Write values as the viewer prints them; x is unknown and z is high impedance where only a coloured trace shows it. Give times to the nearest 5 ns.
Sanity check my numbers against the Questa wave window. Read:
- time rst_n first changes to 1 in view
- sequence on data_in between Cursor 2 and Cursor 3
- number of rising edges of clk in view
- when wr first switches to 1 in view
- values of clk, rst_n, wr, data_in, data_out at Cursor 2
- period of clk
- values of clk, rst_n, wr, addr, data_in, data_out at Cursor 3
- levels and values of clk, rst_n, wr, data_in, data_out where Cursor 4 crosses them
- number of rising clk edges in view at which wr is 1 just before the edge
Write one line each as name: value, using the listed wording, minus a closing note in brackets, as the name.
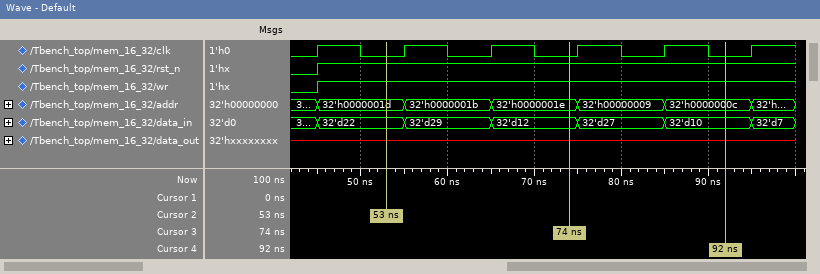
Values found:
time rst_n first changes to 1 in view: 45 ns
sequence on data_in between Cursor 2 and Cursor 3: 32'd22, 32'd29, 32'd12
number of rising edges of clk in view: 6
when wr first switches to 1 in view: 45 ns
values of clk, rst_n, wr, data_in, data_out at Cursor 2: clk=0, rst_n=1, wr=1, data_in=32'd22, data_out=x
period of clk: 10 ns
values of clk, rst_n, wr, addr, data_in, data_out at Cursor 3: clk=0, rst_n=1, wr=1, addr=32'h0000001e, data_in=32'd12, data_out=x
levels and values of clk, rst_n, wr, data_in, data_out where Cursor 4 crosses them: clk=0, rst_n=1, wr=1, data_in=32'd10, data_out=x
number of rising clk edges in view at which wr is 1 just before the edge: 5
